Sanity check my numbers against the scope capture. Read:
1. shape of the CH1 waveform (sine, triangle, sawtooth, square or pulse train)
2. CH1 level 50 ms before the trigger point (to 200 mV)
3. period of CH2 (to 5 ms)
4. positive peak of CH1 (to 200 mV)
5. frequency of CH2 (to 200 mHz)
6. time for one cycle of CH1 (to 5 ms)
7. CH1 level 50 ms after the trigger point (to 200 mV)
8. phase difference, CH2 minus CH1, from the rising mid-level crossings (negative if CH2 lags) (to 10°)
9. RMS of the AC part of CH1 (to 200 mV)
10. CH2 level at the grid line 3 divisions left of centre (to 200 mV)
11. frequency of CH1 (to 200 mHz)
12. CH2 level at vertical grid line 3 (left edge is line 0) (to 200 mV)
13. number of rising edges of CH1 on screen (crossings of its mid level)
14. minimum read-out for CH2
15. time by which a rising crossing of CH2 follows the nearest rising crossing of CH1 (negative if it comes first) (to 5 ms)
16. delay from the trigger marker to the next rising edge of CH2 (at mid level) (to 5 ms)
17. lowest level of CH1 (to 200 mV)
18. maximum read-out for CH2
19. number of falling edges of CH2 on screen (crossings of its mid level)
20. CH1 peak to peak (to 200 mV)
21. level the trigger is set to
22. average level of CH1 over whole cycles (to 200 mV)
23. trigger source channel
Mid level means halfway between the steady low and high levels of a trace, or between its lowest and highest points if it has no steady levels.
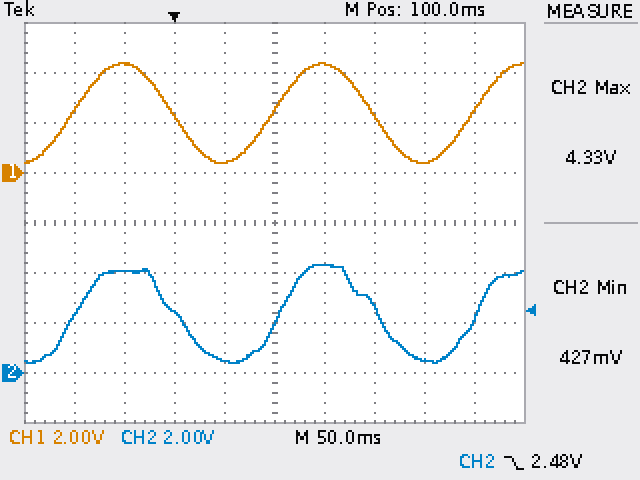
sine
4.4 V
200 ms
4.4 V
5.0 Hz
200 ms
400 mV
-10°
1.4 V
4.0 V
5.0 Hz
2.4 V
3
427 mV
+5 ms
105 ms
400 mV
4.33 V
2
4.0 V
2.48 V
2.4 V
CH2
